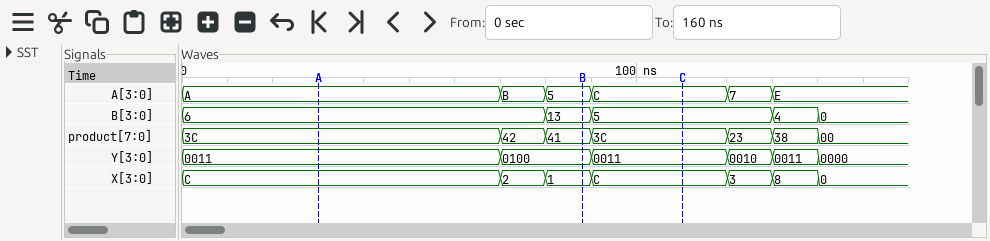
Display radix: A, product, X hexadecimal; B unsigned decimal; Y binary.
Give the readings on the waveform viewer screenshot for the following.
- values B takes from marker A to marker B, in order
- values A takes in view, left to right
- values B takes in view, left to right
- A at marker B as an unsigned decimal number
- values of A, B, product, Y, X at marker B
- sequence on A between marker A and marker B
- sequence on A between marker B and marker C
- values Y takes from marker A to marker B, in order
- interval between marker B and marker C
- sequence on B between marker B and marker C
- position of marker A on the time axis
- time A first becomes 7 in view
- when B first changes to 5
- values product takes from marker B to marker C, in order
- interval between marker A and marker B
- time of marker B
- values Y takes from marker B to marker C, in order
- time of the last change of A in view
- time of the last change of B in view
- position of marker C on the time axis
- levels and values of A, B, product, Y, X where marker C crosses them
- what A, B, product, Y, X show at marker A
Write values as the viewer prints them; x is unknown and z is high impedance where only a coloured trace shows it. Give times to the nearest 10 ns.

6, 13
A, B, 5, C, 7, E
6, 13, 5, 4, 0
5
A=5, B=13, product=41, Y=0100, X=1
A, B, 5
5, C
0011, 0100
20 ns
13, 5
30 ns
120 ns
90 ns
41, 3C
60 ns
90 ns
0100, 0011
130 ns
140 ns
110 ns
A=C, B=5, product=3C, Y=0011, X=C
A=A, B=6, product=3C, Y=0011, X=C
